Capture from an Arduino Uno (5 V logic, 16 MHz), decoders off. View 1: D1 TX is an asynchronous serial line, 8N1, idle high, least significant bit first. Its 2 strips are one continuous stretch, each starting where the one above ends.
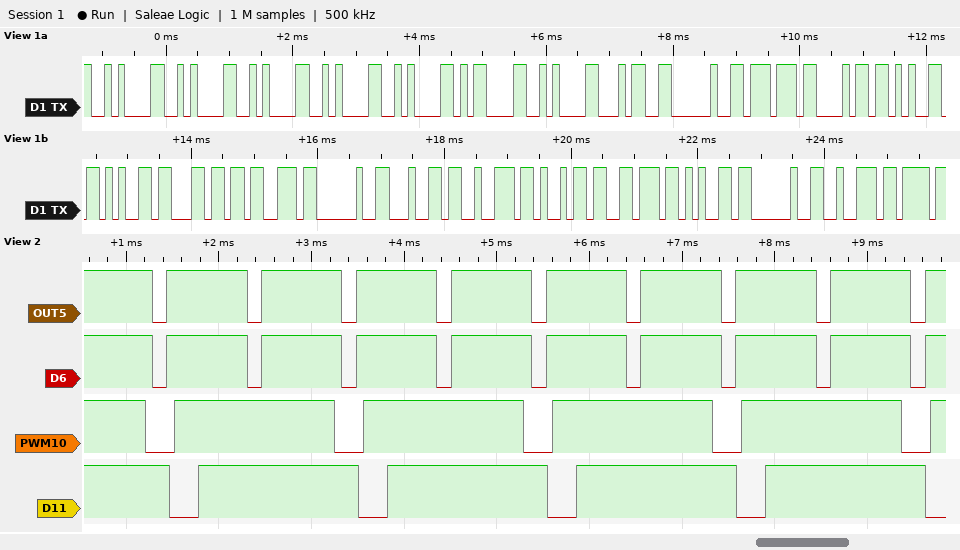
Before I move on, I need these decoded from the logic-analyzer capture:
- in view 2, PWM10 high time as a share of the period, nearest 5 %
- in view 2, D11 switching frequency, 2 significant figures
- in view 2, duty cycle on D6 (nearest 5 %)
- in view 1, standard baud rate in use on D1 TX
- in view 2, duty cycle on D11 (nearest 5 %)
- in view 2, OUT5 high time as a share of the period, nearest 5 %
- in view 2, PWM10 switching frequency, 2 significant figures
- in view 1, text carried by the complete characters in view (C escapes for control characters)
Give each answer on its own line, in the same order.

85 %
490 Hz
85 %
9600 baud
85 %
85 %
490 Hz
"\n\n\n\n\n\r\n4 wheels drive r"
